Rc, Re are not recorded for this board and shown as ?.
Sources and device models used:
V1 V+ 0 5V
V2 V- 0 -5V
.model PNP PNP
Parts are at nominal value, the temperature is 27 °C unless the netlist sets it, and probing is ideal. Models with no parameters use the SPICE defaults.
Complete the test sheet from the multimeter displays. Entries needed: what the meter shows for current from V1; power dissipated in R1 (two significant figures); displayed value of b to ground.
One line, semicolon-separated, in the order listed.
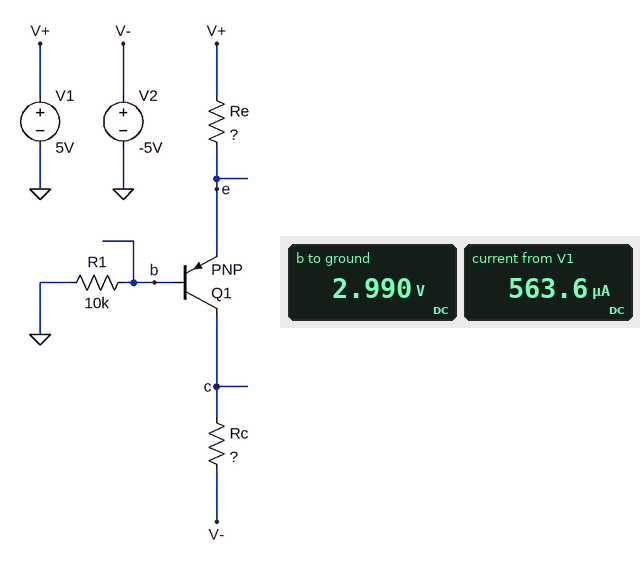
563.6 µA; 890 µW; 2.990 V
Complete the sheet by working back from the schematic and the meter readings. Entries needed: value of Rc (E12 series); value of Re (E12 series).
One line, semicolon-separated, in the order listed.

33 kΩ; 2.2 kΩ
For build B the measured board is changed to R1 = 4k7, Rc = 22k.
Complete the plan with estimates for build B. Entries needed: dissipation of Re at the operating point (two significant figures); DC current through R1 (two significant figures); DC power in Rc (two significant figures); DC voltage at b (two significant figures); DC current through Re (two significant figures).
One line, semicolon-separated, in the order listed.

1.6 mW; 490 µA; 3.0 mW; 2.3 V; 860 µA
